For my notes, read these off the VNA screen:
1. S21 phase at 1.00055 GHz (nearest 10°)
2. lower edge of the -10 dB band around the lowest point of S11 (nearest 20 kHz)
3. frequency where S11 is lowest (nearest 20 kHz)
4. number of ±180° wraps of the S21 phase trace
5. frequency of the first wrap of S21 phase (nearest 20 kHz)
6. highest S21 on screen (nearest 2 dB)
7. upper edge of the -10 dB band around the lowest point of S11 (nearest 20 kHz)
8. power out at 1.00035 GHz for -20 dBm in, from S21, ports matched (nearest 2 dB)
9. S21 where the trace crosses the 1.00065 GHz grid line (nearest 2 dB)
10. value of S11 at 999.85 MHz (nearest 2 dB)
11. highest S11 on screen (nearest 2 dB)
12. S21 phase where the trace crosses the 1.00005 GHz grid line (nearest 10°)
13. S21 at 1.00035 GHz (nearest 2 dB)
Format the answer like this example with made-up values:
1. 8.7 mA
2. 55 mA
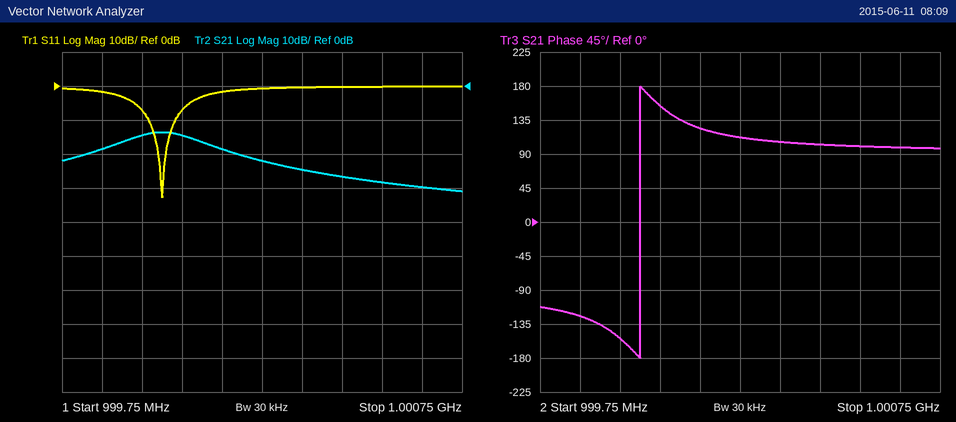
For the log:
1. 100°
2. 999.96 MHz
3. 1.00000 GHz
4. 1
5. 1.00000 GHz
6. -14 dB
7. 1.00004 GHz
8. -44 dBm
9. -30 dB
10. -2 dB
11. 0 dB
12. 150°
13. -24 dB
